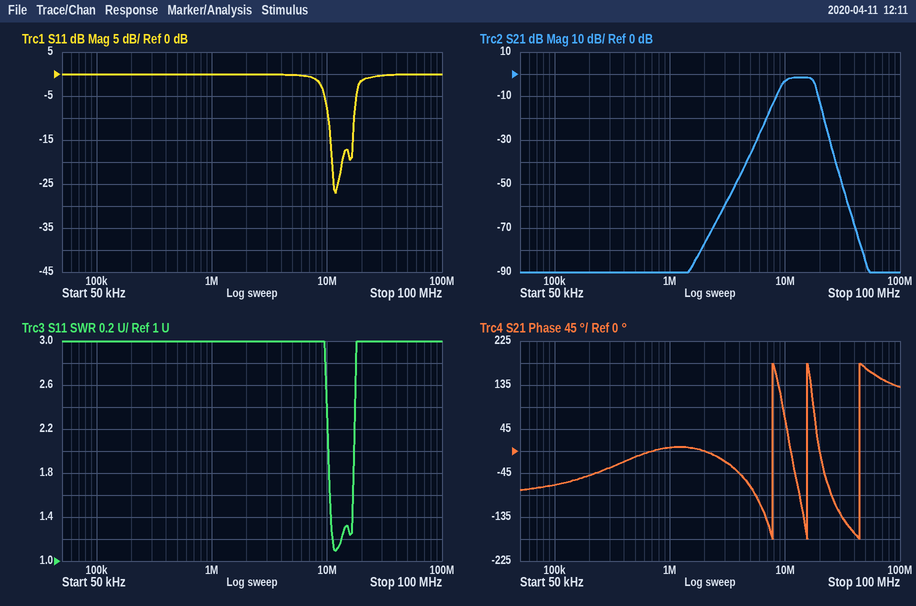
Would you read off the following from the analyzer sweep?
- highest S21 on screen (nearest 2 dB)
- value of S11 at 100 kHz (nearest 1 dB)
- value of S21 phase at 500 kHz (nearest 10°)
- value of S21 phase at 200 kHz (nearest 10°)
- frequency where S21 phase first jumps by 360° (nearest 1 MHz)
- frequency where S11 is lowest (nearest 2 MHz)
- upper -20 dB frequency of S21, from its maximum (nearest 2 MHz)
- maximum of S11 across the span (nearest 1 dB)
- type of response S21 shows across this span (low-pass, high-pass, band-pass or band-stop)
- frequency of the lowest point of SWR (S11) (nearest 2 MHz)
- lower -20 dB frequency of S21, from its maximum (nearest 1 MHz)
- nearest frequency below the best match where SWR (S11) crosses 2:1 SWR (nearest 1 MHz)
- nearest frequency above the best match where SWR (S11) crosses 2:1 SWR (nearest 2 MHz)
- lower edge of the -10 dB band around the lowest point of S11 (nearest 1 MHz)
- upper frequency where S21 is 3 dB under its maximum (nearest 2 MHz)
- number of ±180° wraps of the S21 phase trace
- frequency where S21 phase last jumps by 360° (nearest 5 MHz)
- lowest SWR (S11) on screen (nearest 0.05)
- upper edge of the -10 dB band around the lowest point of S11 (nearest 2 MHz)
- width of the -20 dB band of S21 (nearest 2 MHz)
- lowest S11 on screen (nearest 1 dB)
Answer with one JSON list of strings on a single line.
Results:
["-2 dB", "0 dB", "-10°", "-50°", "8 MHz", "12 MHz", "22 MHz", "0 dB", "band-pass", "12 MHz", "7 MHz", "10 MHz", "18 MHz", "10 MHz", "18 MHz", "3", "45 MHz", "1.10", "18 MHz", "16 MHz", "-27 dB"]
